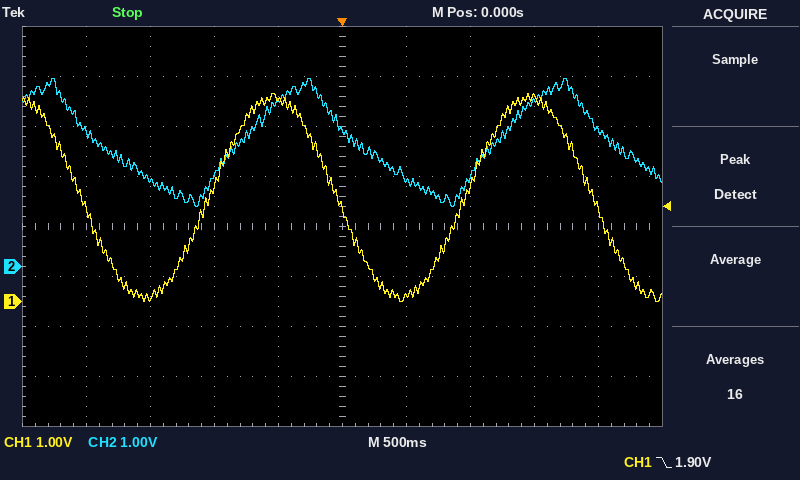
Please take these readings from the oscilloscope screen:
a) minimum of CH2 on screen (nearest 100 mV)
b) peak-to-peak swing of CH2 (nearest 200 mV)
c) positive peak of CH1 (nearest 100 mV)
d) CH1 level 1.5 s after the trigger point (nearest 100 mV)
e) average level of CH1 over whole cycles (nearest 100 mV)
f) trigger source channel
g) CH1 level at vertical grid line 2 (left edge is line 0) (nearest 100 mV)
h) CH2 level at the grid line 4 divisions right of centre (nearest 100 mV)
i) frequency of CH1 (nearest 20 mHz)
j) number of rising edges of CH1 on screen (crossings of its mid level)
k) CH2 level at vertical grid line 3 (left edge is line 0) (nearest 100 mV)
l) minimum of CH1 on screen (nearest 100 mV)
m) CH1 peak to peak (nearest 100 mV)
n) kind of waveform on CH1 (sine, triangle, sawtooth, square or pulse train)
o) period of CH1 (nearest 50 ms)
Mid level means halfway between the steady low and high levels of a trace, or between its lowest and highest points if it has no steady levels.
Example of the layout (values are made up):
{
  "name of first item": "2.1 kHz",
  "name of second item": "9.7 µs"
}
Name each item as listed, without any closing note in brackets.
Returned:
{
  "minimum of CH2 on screen": "1.2 V",
  "peak-to-peak swing of CH2": "2.6 V",
  "positive peak of CH1": "4.2 V",
  "CH1 level 1.5 s after the trigger point": "4.1 V",
  "average level of CH1 over whole cycles": "2.1 V",
  "trigger source channel": "CH1",
  "CH1 level at vertical grid line 2 (left edge is line 0)": "100 mV",
  "CH2 level at the grid line 4 divisions right of centre": "2.7 V",
  "frequency of CH1": "500 mHz",
  "number of rising edges of CH1 on screen": "2",
  "CH2 level at vertical grid line 3 (left edge is line 0)": "1.8 V",
  "minimum of CH1 on screen": "0.0 V",
  "CH1 peak to peak": "4.2 V",
  "kind of waveform on CH1": "sine",
  "period of CH1": "2.00 s"
}
